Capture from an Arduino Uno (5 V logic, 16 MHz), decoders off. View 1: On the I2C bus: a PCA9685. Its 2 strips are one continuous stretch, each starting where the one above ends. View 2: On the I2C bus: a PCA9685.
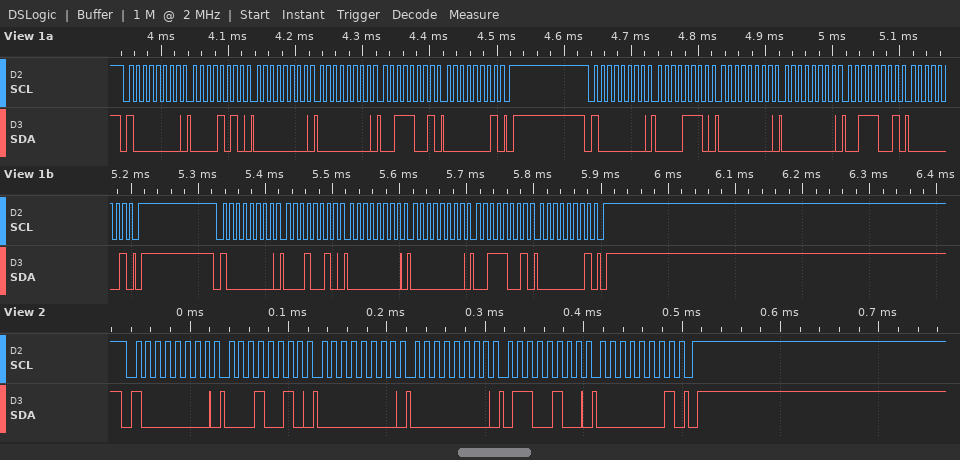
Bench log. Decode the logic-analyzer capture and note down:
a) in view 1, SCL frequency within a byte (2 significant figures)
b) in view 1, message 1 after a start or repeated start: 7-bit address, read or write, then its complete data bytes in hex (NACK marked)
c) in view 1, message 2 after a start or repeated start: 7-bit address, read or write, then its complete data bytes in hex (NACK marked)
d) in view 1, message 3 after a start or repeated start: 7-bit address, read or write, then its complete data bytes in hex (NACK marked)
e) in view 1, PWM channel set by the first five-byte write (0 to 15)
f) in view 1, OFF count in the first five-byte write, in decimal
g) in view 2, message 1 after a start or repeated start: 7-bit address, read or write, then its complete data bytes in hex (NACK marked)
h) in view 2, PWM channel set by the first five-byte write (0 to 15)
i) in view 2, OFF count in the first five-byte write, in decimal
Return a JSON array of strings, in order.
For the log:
["100 kHz", "0x40 write: 0A 00 00 39 01", "0x40 write: 0E 00 00 39 01", "0x40 write: 12 00 00 39 01", "1", "313", "0x40 write: 12 00 00 64 01", "3", "356"]
